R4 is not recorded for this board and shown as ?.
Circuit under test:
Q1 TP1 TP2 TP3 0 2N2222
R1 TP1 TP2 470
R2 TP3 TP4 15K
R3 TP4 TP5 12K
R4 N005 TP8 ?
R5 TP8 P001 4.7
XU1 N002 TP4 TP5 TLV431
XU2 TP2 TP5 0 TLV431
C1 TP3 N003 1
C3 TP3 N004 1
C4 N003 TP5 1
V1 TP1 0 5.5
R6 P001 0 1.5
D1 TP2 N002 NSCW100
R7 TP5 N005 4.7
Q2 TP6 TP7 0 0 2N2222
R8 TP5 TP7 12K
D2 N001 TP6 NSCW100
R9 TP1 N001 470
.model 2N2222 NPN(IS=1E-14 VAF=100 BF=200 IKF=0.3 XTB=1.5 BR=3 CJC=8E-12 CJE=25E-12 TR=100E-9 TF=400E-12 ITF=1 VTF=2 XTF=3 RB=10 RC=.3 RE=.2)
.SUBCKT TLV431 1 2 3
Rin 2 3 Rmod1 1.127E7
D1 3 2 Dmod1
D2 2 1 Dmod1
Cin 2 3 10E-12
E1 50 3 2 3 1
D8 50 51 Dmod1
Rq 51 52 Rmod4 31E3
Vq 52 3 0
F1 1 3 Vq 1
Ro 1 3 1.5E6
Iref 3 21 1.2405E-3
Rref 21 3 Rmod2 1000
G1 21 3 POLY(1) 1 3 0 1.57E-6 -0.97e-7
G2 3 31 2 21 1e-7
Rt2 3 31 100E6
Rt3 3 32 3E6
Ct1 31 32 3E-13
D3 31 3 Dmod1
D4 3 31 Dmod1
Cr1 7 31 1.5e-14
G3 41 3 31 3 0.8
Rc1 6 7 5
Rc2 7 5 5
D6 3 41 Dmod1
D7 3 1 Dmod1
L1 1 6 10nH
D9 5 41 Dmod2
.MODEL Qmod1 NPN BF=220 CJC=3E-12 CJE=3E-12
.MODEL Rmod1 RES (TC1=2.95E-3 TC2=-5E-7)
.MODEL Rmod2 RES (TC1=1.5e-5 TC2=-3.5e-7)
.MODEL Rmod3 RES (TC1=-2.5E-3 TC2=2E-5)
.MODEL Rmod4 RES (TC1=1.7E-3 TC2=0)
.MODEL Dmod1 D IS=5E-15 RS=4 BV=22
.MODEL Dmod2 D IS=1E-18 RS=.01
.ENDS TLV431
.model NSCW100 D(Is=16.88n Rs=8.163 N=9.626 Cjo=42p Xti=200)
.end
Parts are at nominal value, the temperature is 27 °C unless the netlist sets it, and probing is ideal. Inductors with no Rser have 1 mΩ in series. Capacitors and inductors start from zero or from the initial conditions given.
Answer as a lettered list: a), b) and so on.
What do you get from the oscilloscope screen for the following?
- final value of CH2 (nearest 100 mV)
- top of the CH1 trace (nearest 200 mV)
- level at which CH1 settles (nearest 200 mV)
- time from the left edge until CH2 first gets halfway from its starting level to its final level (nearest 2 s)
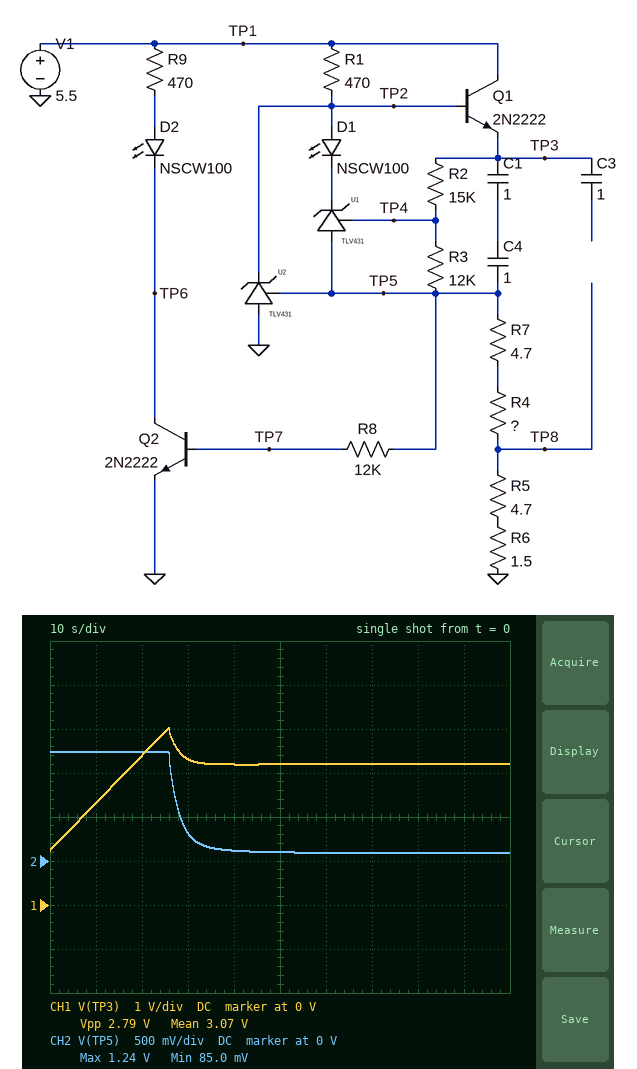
a) 100 mV
b) 4.0 V
c) 3.2 V
d) 28 s
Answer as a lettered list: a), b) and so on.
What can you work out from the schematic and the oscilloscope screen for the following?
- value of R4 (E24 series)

a) 12 Ω
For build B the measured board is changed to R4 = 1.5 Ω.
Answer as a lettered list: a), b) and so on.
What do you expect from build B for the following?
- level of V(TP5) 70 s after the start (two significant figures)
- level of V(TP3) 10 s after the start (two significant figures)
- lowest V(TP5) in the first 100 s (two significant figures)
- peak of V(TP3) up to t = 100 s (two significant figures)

a) 49 mV
b) 3.2 V
c) 48 mV
d) 4.0 V
